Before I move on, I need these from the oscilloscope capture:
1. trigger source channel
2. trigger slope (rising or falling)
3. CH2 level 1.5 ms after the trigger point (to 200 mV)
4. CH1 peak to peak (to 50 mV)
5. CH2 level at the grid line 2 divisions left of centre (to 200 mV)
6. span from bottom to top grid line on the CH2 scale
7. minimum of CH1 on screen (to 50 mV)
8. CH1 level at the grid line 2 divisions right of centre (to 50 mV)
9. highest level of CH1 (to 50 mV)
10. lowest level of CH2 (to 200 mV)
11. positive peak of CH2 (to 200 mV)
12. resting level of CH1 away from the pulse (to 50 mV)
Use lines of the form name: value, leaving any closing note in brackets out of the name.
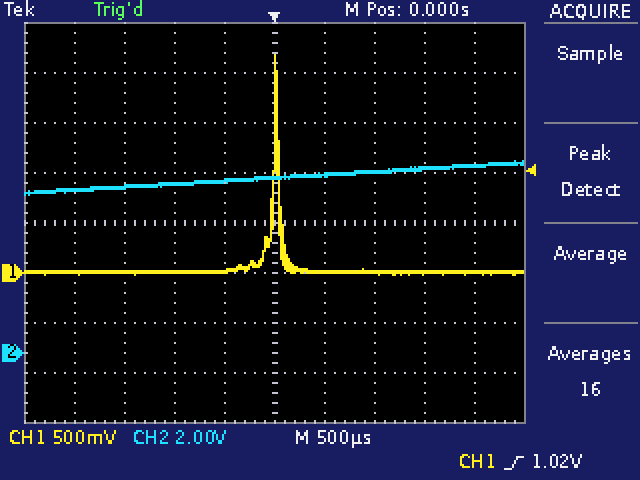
trigger source channel: CH1
trigger slope: rising
CH2 level 1.5 ms after the trigger point: 7.4 V
CH1 peak to peak: 2.20 V
CH2 level at the grid line 2 divisions left of centre: 6.8 V
span from bottom to top grid line on the CH2 scale: 16 V
minimum of CH1 on screen: 0 mV
CH1 level at the grid line 2 divisions right of centre: 0 mV
highest level of CH1: 2.20 V
lowest level of CH2: 6.4 V
positive peak of CH2: 7.6 V
resting level of CH1 away from the pulse: 0 mV
